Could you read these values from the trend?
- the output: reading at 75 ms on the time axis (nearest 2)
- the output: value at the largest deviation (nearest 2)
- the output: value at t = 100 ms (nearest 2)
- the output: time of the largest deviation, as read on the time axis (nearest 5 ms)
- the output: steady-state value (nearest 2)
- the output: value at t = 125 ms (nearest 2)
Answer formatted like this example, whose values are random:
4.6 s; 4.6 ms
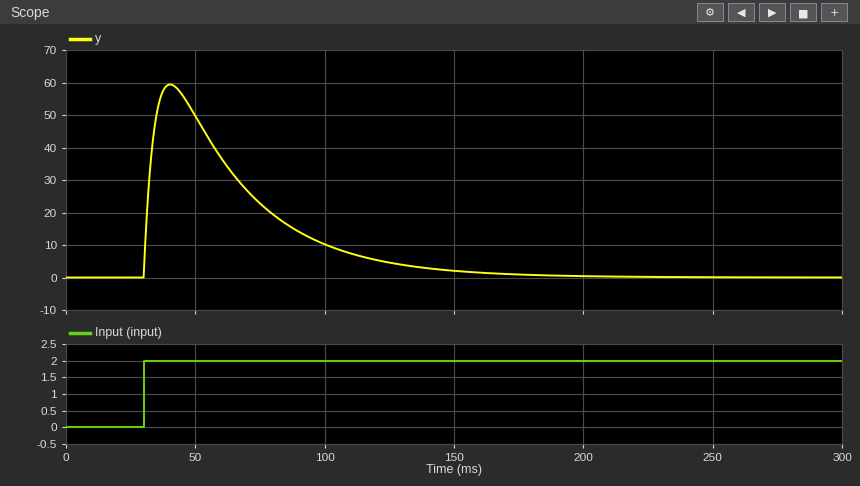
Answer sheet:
22; 60; 10; 40 ms; 0; 4
